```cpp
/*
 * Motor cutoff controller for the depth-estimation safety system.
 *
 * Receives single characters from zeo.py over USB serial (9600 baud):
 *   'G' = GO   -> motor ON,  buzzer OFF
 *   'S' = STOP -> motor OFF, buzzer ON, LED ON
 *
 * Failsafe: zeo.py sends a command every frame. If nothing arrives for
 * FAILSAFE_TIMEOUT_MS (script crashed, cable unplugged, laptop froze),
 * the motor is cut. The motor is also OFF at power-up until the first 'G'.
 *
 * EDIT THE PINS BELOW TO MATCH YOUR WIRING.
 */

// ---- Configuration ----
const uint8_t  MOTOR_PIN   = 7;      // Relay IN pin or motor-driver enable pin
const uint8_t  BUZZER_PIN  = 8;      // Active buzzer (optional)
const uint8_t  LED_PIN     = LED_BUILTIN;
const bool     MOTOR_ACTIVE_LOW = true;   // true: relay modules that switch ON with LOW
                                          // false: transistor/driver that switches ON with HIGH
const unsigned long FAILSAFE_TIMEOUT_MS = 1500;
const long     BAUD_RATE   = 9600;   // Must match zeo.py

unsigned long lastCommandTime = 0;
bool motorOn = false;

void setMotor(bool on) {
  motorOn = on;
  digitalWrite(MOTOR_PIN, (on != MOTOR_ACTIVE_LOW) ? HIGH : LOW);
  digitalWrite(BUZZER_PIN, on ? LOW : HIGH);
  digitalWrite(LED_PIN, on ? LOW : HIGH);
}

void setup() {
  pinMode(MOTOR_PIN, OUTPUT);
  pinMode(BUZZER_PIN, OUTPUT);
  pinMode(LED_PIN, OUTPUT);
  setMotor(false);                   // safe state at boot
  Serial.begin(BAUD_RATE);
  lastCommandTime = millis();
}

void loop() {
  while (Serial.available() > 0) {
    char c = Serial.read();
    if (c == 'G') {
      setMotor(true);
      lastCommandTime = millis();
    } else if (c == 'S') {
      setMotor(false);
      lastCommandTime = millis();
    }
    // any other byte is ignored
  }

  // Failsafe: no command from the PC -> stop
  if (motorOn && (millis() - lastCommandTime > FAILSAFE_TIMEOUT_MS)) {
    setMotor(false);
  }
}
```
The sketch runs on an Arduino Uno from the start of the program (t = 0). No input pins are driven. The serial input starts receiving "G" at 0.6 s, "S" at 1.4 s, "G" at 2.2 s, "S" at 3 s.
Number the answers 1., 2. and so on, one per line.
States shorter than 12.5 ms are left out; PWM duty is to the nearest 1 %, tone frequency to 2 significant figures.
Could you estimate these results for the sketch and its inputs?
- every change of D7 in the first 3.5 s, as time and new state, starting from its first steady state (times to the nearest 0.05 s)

1. 0 s high; 0.6 s low; 1.4 s high; 2.2 s low; 3 s high
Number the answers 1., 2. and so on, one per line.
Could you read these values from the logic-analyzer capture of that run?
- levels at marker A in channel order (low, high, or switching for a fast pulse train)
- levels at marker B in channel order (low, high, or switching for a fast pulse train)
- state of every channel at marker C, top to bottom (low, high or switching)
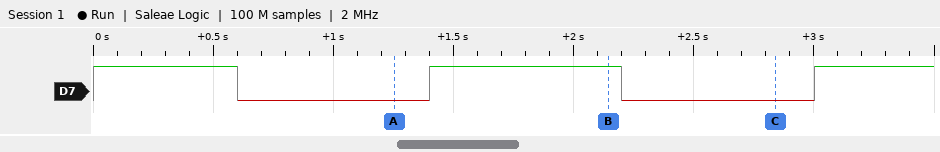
1. D7 low
2. D7 high
3. D7 low
